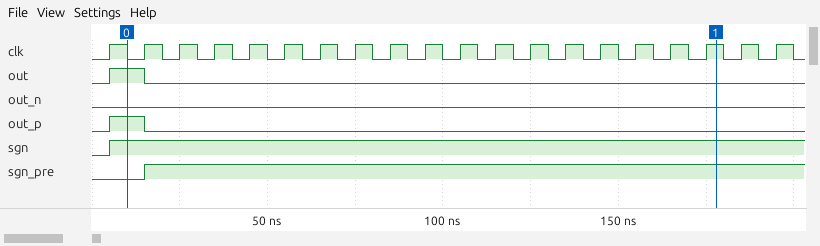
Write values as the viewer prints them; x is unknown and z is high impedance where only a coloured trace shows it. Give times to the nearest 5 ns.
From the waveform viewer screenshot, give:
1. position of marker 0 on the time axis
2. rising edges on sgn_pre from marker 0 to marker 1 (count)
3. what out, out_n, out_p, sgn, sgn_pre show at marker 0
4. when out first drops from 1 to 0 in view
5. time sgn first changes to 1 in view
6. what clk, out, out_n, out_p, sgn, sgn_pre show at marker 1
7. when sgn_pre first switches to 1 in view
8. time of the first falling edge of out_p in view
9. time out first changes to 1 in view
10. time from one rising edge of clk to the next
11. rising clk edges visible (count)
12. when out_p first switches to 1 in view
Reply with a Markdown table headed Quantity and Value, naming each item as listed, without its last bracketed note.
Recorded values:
| Quantity | Value |
|---|---|
| position of marker 0 on the time axis | 10 ns |
| rising edges on sgn_pre from marker 0 to marker 1 | 1 |
| what out, out_n, out_p, sgn, sgn_pre show at marker 0 | out=1, out_n=0, out_p=1, sgn=1, sgn_pre=0 |
| when out first drops from 1 to 0 in view | 15 ns |
| time sgn first changes to 1 in view | 5 ns |
| what clk, out, out_n, out_p, sgn, sgn_pre show at marker 1 | clk=1, out=0, out_n=0, out_p=0, sgn=1, sgn_pre=1 |
| when sgn_pre first switches to 1 in view | 15 ns |
| time of the first falling edge of out_p in view | 15 ns |
| time out first changes to 1 in view | 5 ns |
| time from one rising edge of clk to the next | 10 ns |
| rising clk edges visible | 20 |
| when out_p first switches to 1 in view | 5 ns |
